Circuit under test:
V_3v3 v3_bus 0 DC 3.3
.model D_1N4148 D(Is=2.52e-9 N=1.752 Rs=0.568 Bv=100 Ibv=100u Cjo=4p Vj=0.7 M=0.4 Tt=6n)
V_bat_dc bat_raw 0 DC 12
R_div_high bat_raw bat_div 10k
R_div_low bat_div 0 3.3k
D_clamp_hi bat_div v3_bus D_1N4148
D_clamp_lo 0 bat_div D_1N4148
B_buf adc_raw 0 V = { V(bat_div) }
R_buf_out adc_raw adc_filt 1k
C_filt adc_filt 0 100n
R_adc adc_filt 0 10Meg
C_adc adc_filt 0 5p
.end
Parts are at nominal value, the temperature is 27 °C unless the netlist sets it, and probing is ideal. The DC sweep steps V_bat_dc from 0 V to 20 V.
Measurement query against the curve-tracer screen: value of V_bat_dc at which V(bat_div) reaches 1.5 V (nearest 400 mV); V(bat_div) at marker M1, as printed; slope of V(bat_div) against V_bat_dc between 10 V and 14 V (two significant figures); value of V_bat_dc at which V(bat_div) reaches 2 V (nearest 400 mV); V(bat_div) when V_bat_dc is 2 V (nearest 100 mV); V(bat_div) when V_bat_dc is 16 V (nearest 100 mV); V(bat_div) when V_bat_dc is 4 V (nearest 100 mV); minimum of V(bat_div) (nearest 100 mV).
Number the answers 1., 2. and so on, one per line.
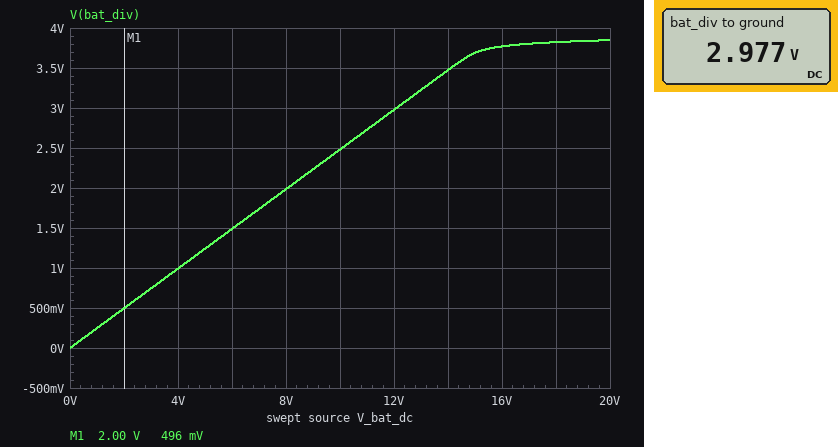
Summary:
1. 6.0 V
2. 496 mV
3. 0.25 V/V
4. 8.0 V
5. 500 mV
6. 3.8 V
7. 1.0 V
8. 0 V
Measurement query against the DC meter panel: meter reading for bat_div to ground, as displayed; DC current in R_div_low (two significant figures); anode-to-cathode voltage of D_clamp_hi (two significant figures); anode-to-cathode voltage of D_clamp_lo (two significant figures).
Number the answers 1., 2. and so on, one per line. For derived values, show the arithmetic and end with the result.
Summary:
1. 2.977 V
2. (2.977 V) / 3.3 kΩ = 900 µA
3. 2.977 V - 3.3 V = -320 mV
4. 0 V - 2.977 V = -3.0 V
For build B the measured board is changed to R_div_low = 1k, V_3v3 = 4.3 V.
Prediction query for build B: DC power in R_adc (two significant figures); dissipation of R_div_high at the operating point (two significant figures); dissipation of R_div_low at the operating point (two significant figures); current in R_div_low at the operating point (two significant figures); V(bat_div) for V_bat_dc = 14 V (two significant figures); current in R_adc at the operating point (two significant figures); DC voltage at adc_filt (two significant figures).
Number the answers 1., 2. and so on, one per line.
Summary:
1. 120 nW
2. 12 mW
3. 1.2 mW
4. 1.1 mA
5. 1.3 V
6. 110 nA
7. 1.1 V
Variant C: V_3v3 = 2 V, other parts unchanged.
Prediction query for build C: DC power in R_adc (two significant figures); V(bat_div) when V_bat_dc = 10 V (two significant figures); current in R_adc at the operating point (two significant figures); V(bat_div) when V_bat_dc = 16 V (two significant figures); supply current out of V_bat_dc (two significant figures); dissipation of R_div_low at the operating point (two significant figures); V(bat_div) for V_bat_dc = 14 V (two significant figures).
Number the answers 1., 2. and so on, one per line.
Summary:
1. 630 nW
2. 2.4 V
3. 250 nA
4. 2.6 V
5. 950 µA
6. 1.9 mW
7. 2.5 V
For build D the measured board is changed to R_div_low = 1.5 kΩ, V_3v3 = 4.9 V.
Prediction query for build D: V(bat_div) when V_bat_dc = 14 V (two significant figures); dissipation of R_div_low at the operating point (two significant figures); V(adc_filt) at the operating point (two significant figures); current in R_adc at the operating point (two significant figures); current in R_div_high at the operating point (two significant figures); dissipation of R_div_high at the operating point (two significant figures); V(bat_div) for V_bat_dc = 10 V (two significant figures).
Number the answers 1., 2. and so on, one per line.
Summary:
1. 1.8 V
2. 1.6 mW
3. 1.6 V
4. 160 nA
5. 1.0 mA
6. 11 mW
7. 1.3 V
